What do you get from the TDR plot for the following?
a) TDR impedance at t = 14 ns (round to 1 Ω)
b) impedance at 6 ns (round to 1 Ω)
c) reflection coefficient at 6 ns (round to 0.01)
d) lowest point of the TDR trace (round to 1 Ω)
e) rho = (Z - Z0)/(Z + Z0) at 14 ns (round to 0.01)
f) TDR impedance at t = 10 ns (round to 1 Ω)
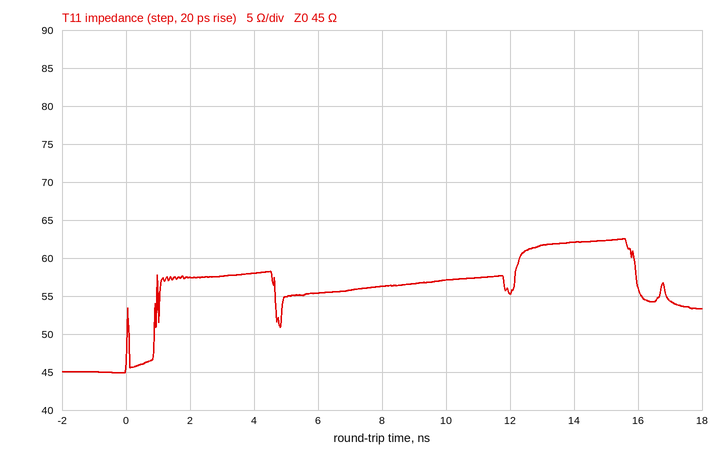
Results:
62 Ω
55 Ω
+0.10
45 Ω
+0.16
57 Ω
